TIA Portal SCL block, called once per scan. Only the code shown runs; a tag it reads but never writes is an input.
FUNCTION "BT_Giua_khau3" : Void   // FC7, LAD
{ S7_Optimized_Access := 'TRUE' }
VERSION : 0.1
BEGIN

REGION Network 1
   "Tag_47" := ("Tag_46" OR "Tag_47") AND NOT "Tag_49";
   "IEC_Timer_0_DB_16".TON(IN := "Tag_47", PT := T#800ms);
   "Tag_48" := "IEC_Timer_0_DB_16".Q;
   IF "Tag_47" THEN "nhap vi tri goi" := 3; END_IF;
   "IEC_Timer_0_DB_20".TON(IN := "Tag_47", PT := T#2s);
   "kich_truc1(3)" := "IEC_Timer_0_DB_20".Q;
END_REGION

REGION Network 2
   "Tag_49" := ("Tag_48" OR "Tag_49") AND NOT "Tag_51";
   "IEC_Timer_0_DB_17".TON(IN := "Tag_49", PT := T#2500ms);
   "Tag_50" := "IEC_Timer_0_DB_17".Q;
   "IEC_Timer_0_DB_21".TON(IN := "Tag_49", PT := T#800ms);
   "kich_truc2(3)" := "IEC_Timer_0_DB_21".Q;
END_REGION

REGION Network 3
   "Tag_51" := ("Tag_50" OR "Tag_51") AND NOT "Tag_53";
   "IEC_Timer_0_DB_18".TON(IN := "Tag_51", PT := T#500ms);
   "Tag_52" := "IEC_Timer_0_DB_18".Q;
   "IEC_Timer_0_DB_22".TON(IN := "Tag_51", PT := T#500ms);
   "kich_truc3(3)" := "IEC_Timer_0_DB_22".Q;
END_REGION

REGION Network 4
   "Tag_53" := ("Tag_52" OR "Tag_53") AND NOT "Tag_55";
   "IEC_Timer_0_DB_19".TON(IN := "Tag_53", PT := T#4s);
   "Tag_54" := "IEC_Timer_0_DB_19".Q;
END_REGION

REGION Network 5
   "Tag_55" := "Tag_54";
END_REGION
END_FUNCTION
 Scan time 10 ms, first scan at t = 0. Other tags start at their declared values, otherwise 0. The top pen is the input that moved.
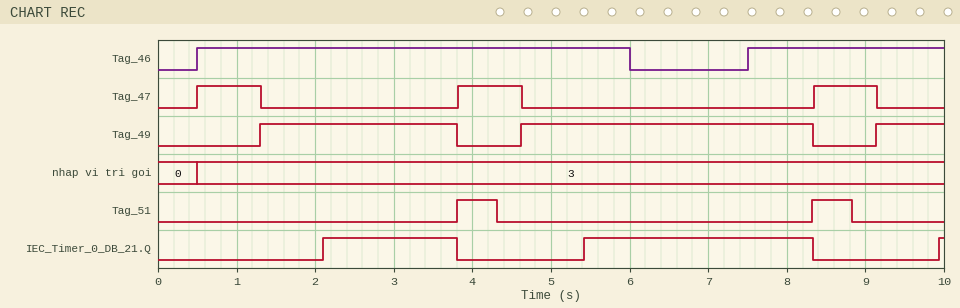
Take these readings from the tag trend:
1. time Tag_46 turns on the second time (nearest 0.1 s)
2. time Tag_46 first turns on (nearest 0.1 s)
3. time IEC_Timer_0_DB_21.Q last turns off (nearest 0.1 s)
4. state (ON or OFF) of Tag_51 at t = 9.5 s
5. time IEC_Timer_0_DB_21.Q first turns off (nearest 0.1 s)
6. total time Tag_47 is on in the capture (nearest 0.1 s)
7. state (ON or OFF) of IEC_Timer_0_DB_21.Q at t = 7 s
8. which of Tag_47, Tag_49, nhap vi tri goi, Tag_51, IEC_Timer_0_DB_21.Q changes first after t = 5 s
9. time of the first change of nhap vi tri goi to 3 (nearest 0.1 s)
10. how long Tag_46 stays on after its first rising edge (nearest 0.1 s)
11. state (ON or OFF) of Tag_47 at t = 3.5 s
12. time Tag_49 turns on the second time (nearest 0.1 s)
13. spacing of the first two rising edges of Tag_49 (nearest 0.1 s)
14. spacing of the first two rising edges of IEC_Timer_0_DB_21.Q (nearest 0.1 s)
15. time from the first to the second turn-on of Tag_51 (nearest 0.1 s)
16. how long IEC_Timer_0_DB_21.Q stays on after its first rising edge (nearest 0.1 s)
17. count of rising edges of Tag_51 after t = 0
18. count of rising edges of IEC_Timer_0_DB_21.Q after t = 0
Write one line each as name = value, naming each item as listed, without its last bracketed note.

time Tag_46 turns on the second time = 7.5 s
time Tag_46 first turns on = 0.5 s
time IEC_Timer_0_DB_21.Q last turns off = 8.3 s
state (ON or OFF) of Tag_51 at t = 9.5 s = OFF
time IEC_Timer_0_DB_21.Q first turns off = 3.8 s
total time Tag_47 is on in the capture = 2.4 s
state (ON or OFF) of IEC_Timer_0_DB_21.Q at t = 7 s = ON
which of Tag_47, Tag_49, nhap vi tri goi, Tag_51, IEC_Timer_0_DB_21.Q changes first after t = 5 s = IEC_Timer_0_DB_21.Q
time of the first change of nhap vi tri goi to 3 = 0.5 s
how long Tag_46 stays on after its first rising edge = 5.5 s
state (ON or OFF) of Tag_47 at t = 3.5 s = OFF
time Tag_49 turns on the second time = 4.6 s
spacing of the first two rising edges of Tag_49 = 3.3 s
spacing of the first two rising edges of IEC_Timer_0_DB_21.Q = 3.3 s
time from the first to the second turn-on of Tag_51 = 4.5 s
how long IEC_Timer_0_DB_21.Q stays on after its first rising edge = 1.7 s
count of rising edges of Tag_51 after t = 0 = 2
count of rising edges of IEC_Timer_0_DB_21.Q after t = 0 = 3
